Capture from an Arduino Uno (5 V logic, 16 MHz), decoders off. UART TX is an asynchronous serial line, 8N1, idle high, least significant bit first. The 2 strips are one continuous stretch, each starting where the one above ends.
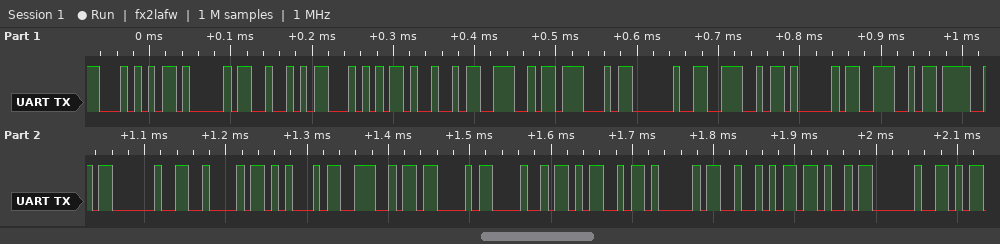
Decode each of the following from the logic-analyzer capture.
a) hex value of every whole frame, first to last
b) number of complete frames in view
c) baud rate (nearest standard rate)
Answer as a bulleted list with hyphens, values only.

- 54 41 52 54 49 4E 47 20 4E 41 4E 4F 20 42 45 4E 43 48 4D 41 52 4B 20
- 23
- 115200 baud
